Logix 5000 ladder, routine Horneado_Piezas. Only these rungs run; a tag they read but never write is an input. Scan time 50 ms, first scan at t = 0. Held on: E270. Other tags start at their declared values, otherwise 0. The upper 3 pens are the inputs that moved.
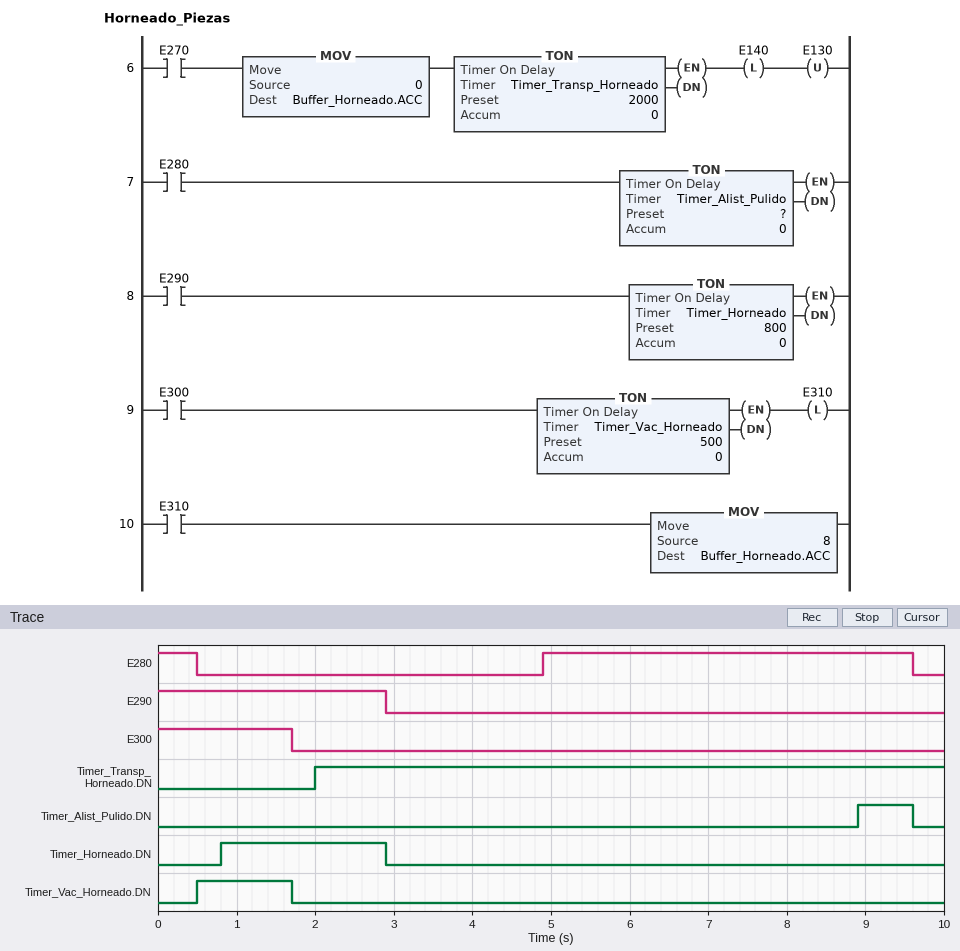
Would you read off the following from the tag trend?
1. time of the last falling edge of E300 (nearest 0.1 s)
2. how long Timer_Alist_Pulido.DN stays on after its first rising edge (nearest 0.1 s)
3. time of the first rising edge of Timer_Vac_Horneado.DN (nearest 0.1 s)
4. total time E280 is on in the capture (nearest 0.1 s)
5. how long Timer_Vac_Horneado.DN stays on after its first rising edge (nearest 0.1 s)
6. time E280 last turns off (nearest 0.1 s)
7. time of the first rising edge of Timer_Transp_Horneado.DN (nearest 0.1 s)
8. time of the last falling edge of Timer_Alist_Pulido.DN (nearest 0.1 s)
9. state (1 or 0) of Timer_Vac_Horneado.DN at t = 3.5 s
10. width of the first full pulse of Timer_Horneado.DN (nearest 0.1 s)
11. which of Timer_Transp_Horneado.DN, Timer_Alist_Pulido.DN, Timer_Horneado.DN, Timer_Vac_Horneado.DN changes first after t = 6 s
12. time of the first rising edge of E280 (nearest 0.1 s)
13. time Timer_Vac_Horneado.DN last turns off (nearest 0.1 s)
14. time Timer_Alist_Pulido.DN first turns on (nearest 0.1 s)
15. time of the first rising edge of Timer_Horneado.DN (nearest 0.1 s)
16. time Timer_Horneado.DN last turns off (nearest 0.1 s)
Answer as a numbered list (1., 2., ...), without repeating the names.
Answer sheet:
1. 1.7 s
2. 0.7 s
3. 0.5 s
4. 5.2 s
5. 1.2 s
6. 9.6 s
7. 2.0 s
8. 9.6 s
9. 0
10. 2.1 s
11. Timer_Alist_Pulido.DN
12. 4.9 s
13. 1.7 s
14. 8.9 s
15. 0.8 s
16. 2.9 s
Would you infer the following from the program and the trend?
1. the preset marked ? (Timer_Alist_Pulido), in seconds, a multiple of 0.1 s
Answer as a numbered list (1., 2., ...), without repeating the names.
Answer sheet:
1. 4.0 s
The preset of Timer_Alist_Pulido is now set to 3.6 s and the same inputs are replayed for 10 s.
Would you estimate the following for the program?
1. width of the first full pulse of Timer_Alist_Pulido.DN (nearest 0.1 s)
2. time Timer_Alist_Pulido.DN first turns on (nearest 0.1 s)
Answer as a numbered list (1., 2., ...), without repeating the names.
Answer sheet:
1. 1.1 s
2. 8.5 s
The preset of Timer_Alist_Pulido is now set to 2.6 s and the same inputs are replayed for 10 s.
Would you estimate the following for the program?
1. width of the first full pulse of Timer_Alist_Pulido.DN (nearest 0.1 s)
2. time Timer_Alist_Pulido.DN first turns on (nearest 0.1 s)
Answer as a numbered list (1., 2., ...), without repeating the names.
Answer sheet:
1. 2.1 s
2. 7.5 s
